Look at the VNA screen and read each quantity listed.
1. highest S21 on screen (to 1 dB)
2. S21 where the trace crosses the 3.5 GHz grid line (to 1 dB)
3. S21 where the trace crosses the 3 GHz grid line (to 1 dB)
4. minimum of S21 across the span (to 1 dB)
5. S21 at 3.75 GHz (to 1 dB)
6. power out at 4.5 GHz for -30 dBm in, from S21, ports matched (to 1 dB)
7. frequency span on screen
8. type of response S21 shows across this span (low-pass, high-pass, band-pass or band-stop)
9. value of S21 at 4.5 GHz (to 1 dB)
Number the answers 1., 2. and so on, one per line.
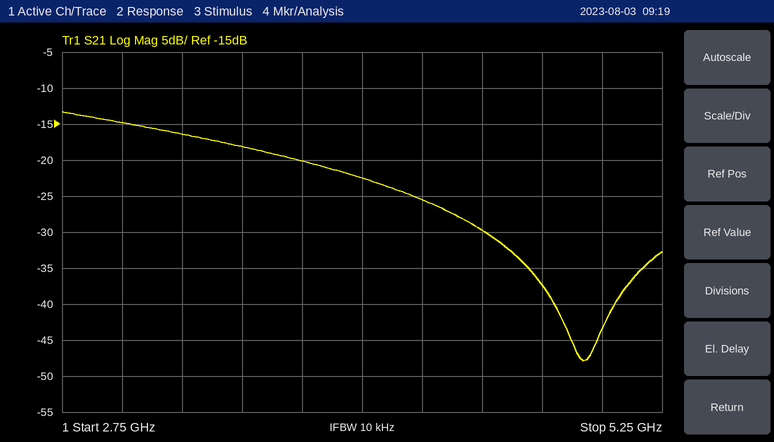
1. -13 dB
2. -18 dB
3. -15 dB
4. -48 dB
5. -20 dB
6. -60 dBm
7. 2.5 GHz
8. low-pass
9. -30 dB
